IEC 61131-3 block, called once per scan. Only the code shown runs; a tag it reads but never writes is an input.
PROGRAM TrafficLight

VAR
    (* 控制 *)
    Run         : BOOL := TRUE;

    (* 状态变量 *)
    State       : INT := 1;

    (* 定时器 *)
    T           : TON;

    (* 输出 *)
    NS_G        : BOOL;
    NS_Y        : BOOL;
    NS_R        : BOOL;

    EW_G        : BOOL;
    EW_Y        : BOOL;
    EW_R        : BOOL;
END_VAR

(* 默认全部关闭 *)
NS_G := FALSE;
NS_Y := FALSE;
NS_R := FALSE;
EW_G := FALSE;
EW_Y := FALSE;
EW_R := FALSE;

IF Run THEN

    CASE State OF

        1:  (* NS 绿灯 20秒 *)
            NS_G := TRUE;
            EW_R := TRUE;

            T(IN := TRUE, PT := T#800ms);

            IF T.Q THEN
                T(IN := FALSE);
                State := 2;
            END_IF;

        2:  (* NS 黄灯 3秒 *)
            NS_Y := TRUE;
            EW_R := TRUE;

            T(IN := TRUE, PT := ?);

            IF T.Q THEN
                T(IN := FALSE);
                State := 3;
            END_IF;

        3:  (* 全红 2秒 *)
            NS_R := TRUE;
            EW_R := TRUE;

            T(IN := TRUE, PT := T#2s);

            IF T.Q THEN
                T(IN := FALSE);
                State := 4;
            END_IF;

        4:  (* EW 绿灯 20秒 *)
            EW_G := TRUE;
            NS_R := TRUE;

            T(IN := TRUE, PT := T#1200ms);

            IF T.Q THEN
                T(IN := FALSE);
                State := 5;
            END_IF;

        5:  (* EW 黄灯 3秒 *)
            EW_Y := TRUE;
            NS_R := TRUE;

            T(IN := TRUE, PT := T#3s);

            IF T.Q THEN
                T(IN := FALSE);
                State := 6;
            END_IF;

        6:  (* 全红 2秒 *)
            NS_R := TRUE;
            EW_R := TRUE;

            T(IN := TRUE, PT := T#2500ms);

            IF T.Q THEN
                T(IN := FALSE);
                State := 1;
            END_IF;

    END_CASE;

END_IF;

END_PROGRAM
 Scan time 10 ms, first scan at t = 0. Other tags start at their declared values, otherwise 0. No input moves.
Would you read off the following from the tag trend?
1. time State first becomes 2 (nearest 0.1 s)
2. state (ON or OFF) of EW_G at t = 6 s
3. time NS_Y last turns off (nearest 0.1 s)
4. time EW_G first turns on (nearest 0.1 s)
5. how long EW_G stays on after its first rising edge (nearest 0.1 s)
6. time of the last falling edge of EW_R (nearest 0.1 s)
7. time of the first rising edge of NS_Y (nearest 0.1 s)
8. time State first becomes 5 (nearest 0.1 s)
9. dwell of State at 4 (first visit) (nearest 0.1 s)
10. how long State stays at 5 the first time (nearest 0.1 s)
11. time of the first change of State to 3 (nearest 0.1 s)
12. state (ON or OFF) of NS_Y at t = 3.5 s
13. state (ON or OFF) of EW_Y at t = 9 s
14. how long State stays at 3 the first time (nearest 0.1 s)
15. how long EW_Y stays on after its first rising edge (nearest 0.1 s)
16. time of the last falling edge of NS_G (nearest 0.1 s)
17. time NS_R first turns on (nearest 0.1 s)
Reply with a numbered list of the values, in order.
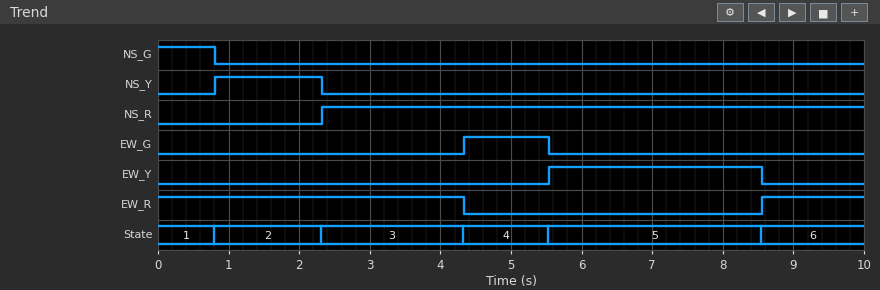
1. 0.8 s
2. OFF
3. 2.3 s
4. 4.3 s
5. 1.2 s
6. 4.3 s
7. 0.8 s
8. 5.5 s
9. 1.2 s
10. 3.0 s
11. 2.3 s
12. OFF
13. OFF
14. 2.0 s
15. 3.0 s
16. 0.8 s
17. 2.3 s
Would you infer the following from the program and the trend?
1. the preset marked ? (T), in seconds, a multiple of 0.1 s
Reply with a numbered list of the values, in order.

1. 1.5 s
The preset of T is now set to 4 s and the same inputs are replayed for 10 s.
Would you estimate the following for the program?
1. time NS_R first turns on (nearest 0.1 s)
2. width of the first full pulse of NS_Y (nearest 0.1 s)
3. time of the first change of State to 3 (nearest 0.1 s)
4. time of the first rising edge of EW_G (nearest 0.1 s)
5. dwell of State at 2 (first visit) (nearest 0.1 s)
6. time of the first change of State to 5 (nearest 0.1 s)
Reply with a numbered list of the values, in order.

1. 4.8 s
2. 4.0 s
3. 4.8 s
4. 6.8 s
5. 4.0 s
6. 8.0 s
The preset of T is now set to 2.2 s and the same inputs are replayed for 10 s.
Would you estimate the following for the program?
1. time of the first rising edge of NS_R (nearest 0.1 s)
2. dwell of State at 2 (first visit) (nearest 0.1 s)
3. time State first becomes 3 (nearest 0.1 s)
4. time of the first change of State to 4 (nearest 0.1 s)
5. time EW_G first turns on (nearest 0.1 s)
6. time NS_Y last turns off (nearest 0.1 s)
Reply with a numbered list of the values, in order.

1. 3.0 s
2. 2.2 s
3. 3.0 s
4. 5.0 s
5. 5.0 s
6. 3.0 s
